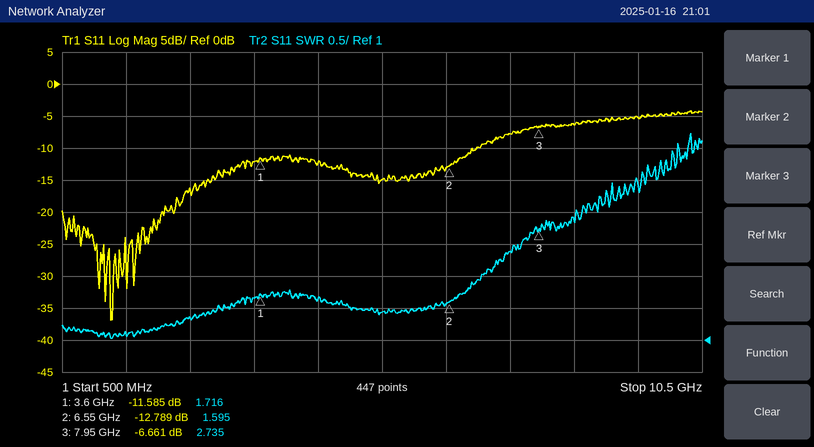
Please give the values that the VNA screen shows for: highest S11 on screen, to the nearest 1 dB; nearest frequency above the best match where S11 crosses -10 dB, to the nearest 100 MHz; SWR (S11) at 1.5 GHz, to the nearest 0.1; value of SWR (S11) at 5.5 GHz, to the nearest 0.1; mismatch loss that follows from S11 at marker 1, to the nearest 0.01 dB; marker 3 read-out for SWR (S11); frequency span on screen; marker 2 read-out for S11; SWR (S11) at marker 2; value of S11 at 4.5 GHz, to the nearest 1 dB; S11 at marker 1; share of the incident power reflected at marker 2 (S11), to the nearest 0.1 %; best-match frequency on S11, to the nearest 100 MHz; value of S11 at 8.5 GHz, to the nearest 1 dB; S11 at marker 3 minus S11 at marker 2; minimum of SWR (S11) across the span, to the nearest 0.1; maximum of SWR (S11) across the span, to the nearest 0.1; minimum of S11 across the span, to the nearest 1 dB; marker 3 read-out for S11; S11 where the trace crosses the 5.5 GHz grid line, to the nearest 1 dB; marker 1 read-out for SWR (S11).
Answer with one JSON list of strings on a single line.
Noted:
["-4 dB", "7.0 GHz", "1.1", "1.4", "0.31 dB", "2.735", "10 GHz", "-12.789 dB", "1.595", "-12 dB", "-11.585 dB", "5.3 %", "1.3 GHz", "-6 dB", "6.128 dB", "1.0", "4.2", "-37 dB", "-6.661 dB", "-15 dB", "1.716"]
